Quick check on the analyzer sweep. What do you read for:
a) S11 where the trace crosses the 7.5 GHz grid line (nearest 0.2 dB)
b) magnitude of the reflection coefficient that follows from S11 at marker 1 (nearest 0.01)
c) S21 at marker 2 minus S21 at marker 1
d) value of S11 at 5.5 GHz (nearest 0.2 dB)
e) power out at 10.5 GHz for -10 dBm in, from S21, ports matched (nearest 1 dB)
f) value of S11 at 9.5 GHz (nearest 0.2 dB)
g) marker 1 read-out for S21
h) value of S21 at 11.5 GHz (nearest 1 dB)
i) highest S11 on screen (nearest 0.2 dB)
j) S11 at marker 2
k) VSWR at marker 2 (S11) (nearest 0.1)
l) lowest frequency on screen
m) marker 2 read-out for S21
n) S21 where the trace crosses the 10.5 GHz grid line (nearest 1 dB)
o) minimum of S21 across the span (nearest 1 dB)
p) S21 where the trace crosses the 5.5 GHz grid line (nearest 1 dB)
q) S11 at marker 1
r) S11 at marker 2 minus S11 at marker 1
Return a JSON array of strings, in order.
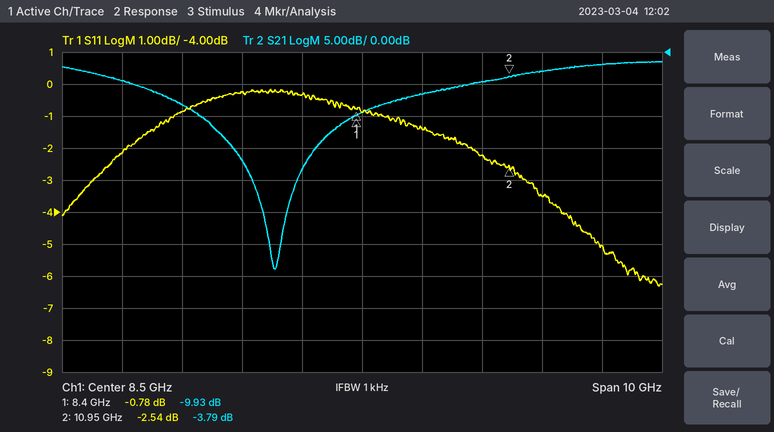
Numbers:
["-0.4 dB", "0.91", "6.14 dB", "-0.8 dB", "-15 dBm", "-1.4 dB", "-9.93 dB", "-3 dB", "-0.2 dB", "-2.54 dB", "6.9", "3.5 GHz", "-3.79 dB", "-5 dB", "-34 dB", "-8 dB", "-0.78 dB", "-1.76 dB"]
